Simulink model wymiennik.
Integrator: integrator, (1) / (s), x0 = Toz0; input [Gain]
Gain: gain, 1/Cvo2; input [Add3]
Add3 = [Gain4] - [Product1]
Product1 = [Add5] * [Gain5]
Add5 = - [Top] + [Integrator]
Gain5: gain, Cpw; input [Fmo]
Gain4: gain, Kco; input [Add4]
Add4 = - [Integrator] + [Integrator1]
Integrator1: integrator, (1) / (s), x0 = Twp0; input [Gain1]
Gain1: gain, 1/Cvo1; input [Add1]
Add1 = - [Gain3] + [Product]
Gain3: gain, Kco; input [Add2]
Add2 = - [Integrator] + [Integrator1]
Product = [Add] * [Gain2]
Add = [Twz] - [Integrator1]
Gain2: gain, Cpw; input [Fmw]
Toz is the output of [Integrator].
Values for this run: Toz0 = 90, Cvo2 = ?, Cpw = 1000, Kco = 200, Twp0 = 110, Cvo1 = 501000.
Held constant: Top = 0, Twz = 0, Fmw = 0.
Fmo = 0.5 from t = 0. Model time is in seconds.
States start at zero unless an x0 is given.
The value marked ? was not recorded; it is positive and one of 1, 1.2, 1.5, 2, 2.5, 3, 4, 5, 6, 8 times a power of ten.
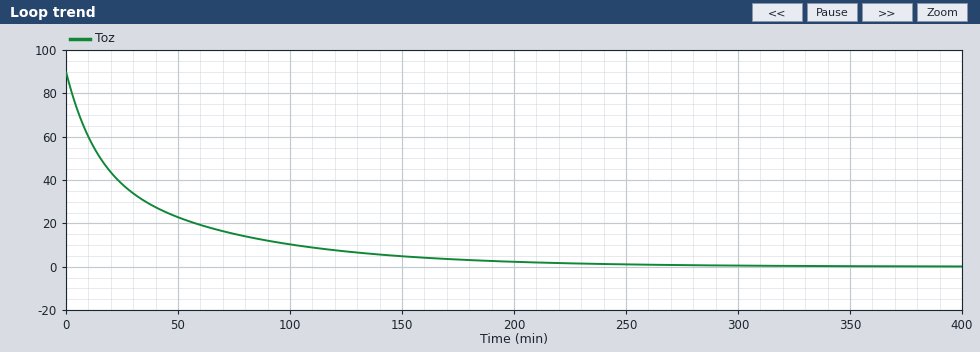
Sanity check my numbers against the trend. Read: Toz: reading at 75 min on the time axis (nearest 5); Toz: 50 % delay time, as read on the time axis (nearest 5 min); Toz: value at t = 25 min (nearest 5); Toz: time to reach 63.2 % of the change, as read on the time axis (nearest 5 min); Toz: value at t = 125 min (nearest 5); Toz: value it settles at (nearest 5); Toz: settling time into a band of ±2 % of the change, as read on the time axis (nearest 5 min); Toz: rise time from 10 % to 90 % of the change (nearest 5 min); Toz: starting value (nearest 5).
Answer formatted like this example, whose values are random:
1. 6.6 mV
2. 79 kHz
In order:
1. 15
2. 20 min
3. 40
4. 30 min
5. 5
6. 0
7. 215 min
8. 105 min
9. 90
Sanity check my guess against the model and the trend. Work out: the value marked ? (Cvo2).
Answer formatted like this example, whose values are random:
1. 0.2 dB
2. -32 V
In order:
1. 600000
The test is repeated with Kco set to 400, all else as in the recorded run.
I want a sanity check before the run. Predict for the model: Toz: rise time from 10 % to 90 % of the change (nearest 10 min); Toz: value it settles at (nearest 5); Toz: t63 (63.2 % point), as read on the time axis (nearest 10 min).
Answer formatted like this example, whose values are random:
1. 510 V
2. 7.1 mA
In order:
1. 100 min
2. 0
3. 40 min
